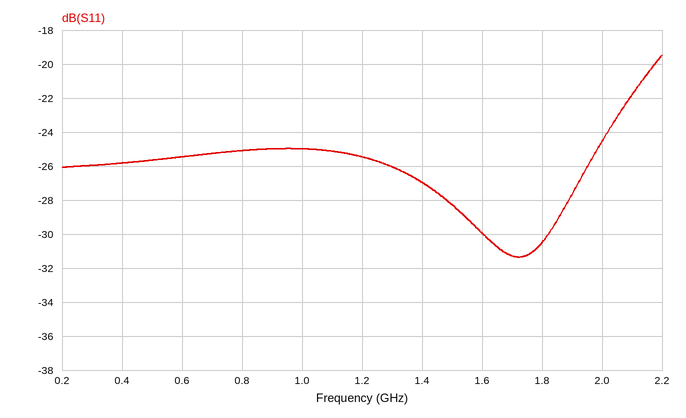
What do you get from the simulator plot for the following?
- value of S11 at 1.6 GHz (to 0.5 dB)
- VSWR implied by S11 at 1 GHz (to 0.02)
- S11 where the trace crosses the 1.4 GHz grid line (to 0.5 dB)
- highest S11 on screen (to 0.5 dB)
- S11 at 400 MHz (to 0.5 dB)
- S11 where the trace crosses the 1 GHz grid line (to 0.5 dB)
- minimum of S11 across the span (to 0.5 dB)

-30.0 dB
1.12
-27.0 dB
-19.5 dB
-26.0 dB
-25.0 dB
-31.5 dB
